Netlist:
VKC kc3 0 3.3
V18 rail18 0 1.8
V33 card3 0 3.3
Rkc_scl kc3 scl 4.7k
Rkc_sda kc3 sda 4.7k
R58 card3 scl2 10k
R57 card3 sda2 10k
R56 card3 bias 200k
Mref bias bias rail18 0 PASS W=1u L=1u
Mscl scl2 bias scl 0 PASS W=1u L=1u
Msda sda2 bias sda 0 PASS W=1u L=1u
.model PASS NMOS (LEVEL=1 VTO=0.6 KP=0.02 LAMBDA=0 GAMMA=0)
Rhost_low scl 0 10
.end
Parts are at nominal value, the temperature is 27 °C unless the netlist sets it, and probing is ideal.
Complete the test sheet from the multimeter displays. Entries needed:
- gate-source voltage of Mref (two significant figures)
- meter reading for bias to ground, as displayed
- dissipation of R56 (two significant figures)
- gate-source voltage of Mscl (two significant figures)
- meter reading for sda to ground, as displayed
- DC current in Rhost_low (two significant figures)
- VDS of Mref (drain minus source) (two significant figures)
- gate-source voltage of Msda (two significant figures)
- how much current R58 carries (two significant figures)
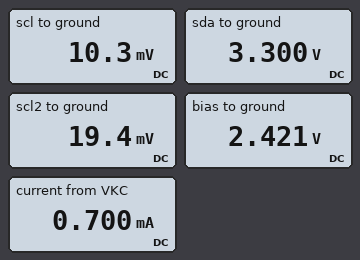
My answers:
620 mV
2.421 V
3.9 µW
2.4 V
3.300 V
1.0 mA
620 mV
-880 mV
330 µA
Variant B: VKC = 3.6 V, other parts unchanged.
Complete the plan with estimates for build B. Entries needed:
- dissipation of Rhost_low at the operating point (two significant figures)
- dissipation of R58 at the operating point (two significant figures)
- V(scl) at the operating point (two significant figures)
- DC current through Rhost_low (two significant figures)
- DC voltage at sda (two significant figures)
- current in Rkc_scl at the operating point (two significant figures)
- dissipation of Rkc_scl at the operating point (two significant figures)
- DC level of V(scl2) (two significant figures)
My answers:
12 µW
1.1 mW
11 mV
1.1 mA
3.6 V
760 µA
2.7 mW
20 mV
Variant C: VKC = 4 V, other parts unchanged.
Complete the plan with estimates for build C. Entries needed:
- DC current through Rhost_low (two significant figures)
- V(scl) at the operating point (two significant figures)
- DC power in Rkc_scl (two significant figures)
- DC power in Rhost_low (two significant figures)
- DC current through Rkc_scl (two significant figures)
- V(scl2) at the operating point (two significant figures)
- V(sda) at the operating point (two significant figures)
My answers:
1.2 mA
12 mV
3.4 mW
14 µW
850 µA
21 mV
4.0 V
